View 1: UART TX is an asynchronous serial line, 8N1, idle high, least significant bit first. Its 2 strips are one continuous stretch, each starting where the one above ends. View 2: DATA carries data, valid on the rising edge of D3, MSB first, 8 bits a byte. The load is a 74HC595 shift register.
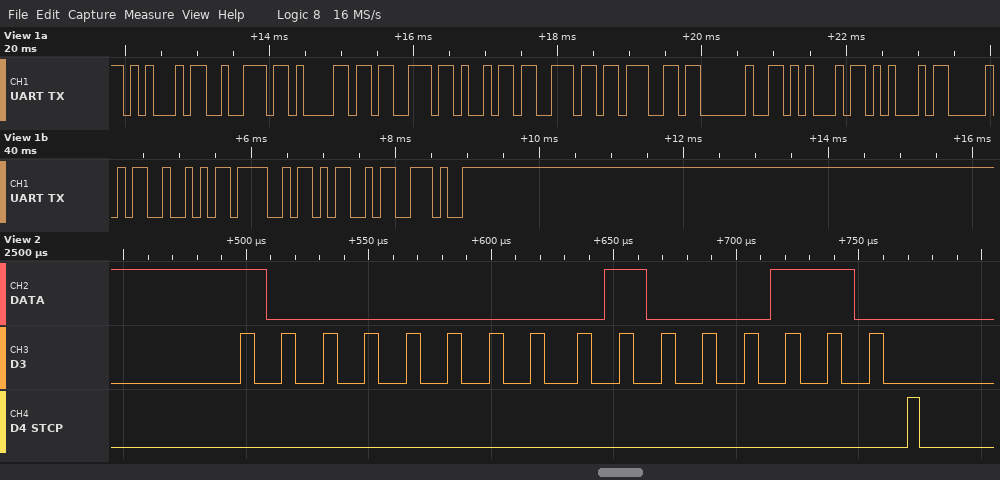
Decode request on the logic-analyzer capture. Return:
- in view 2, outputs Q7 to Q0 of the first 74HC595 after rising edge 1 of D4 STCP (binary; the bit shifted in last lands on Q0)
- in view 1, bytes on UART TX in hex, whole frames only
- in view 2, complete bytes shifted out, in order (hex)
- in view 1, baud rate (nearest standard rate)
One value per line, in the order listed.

01000110
45 72 61 73 69 6E 67 20 45 45 50 52 4F 4D 2E
80 46
9600 baud
